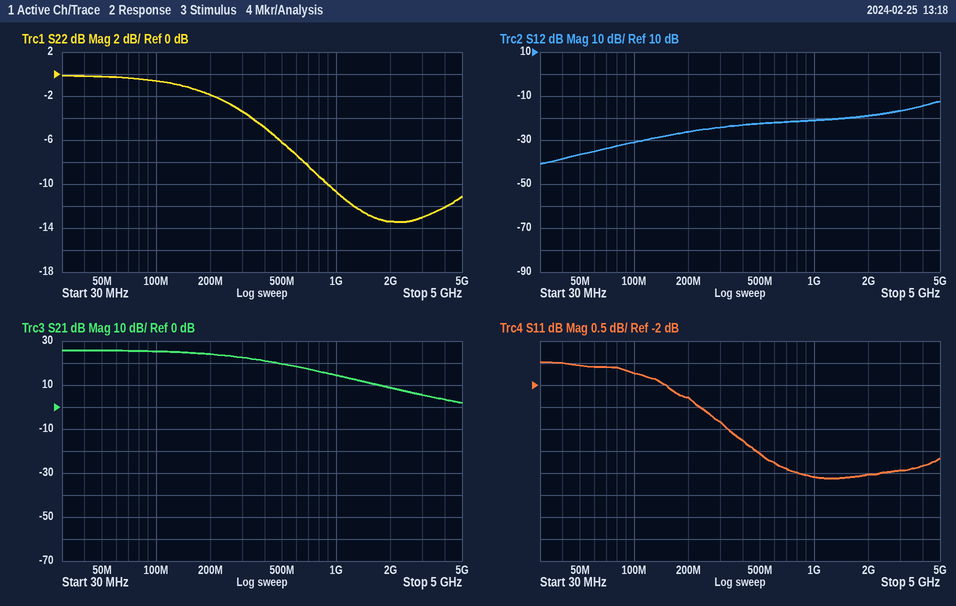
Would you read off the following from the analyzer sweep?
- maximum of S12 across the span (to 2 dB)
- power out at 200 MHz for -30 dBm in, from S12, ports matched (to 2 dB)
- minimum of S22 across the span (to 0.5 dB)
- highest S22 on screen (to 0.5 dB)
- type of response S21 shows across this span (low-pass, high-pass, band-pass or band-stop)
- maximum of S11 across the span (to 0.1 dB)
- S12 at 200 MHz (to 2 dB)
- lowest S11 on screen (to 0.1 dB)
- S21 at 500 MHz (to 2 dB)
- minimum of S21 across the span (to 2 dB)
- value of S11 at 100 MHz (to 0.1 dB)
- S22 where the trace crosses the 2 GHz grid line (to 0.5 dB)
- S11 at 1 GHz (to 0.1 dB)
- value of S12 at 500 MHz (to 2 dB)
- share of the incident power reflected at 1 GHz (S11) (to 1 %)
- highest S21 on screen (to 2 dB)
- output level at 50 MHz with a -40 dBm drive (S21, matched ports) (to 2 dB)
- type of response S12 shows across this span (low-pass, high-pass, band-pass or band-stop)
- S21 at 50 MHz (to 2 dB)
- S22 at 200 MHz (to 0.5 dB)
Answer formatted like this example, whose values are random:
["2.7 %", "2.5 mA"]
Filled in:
["-12 dB", "-56 dBm", "-13.5 dB", "0.0 dB", "low-pass", "-1.5 dB", "-26 dB", "-4.1 dB", "20 dB", "2 dB", "-1.7 dB", "-13.5 dB", "-4.1 dB", "-22 dB", "39 %", "26 dB", "-14 dBm", "high-pass", "26 dB", "-2.0 dB"]
